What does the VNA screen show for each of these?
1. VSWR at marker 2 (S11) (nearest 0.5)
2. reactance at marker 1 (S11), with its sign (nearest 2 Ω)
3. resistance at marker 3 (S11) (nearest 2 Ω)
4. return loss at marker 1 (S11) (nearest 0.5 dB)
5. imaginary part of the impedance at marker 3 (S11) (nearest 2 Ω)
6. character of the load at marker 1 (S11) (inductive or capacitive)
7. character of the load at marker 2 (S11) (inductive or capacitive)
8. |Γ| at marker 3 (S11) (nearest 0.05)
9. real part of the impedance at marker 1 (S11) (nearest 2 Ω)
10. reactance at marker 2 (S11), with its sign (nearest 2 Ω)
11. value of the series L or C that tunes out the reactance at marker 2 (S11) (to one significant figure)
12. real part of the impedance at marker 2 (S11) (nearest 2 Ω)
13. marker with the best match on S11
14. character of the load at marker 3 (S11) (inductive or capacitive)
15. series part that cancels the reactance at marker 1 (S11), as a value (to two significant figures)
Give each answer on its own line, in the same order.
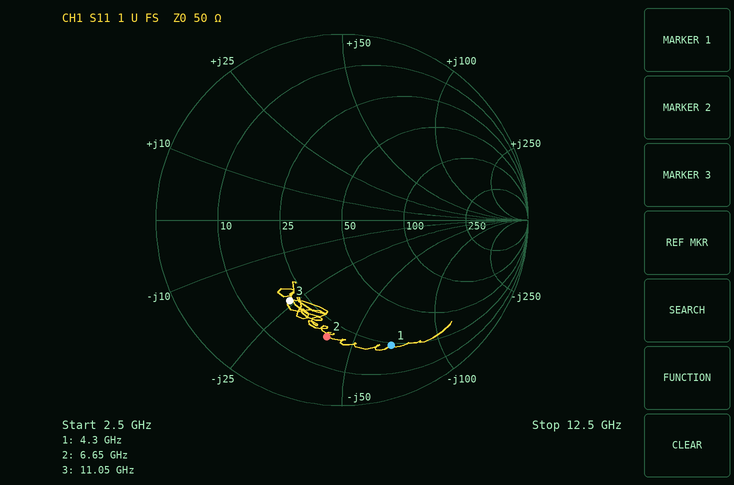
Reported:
4.5
-68 Ω
20 Ω
3.0 dB
-24 Ω
capacitive
capacitive
0.50
24 Ω
-40 Ω
1.0 nH
20 Ω
marker 3
capacitive
2.5 nH
